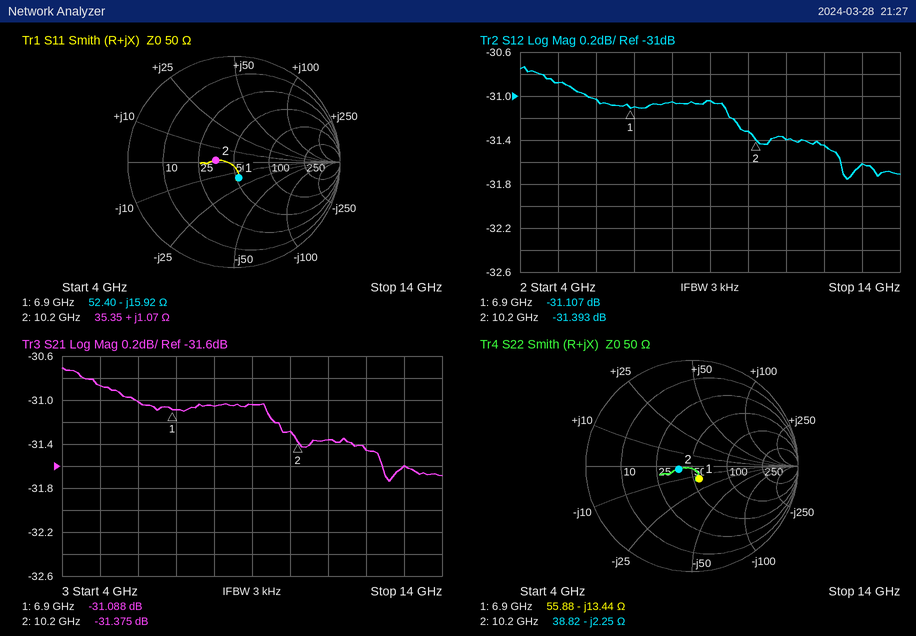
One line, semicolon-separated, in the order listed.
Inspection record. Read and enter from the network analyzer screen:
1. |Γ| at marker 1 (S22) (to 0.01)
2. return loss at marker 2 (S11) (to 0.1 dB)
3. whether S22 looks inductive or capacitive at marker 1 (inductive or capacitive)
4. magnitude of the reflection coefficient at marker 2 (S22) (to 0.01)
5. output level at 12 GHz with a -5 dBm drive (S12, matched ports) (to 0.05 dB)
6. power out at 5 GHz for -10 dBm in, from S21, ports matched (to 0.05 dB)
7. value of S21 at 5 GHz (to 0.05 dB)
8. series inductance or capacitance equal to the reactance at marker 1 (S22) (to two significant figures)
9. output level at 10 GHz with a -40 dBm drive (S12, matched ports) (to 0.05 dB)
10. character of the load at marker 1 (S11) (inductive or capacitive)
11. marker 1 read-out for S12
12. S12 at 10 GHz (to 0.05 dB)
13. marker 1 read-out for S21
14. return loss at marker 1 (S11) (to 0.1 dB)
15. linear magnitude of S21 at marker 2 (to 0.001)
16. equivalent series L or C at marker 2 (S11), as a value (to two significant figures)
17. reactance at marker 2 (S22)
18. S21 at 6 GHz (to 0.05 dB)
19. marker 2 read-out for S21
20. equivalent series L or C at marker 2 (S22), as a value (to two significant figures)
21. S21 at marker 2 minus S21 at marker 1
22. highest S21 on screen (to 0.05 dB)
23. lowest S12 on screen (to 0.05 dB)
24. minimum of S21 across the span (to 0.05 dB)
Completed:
0.14; 15.3 dB; capacitive; 0.13; -36.45 dBm; -40.85 dBm; -30.85 dB; 1.7 pF; -71.30 dBm; capacitive; -31.107 dB; -31.30 dB; -31.088 dB; 16.2 dB; 0.027; 17 pH; -2.25 Ω; -31.00 dB; -31.375 dB; 6.9 pF; -0.287 dB; -30.70 dB; -31.75 dB; -31.75 dB
